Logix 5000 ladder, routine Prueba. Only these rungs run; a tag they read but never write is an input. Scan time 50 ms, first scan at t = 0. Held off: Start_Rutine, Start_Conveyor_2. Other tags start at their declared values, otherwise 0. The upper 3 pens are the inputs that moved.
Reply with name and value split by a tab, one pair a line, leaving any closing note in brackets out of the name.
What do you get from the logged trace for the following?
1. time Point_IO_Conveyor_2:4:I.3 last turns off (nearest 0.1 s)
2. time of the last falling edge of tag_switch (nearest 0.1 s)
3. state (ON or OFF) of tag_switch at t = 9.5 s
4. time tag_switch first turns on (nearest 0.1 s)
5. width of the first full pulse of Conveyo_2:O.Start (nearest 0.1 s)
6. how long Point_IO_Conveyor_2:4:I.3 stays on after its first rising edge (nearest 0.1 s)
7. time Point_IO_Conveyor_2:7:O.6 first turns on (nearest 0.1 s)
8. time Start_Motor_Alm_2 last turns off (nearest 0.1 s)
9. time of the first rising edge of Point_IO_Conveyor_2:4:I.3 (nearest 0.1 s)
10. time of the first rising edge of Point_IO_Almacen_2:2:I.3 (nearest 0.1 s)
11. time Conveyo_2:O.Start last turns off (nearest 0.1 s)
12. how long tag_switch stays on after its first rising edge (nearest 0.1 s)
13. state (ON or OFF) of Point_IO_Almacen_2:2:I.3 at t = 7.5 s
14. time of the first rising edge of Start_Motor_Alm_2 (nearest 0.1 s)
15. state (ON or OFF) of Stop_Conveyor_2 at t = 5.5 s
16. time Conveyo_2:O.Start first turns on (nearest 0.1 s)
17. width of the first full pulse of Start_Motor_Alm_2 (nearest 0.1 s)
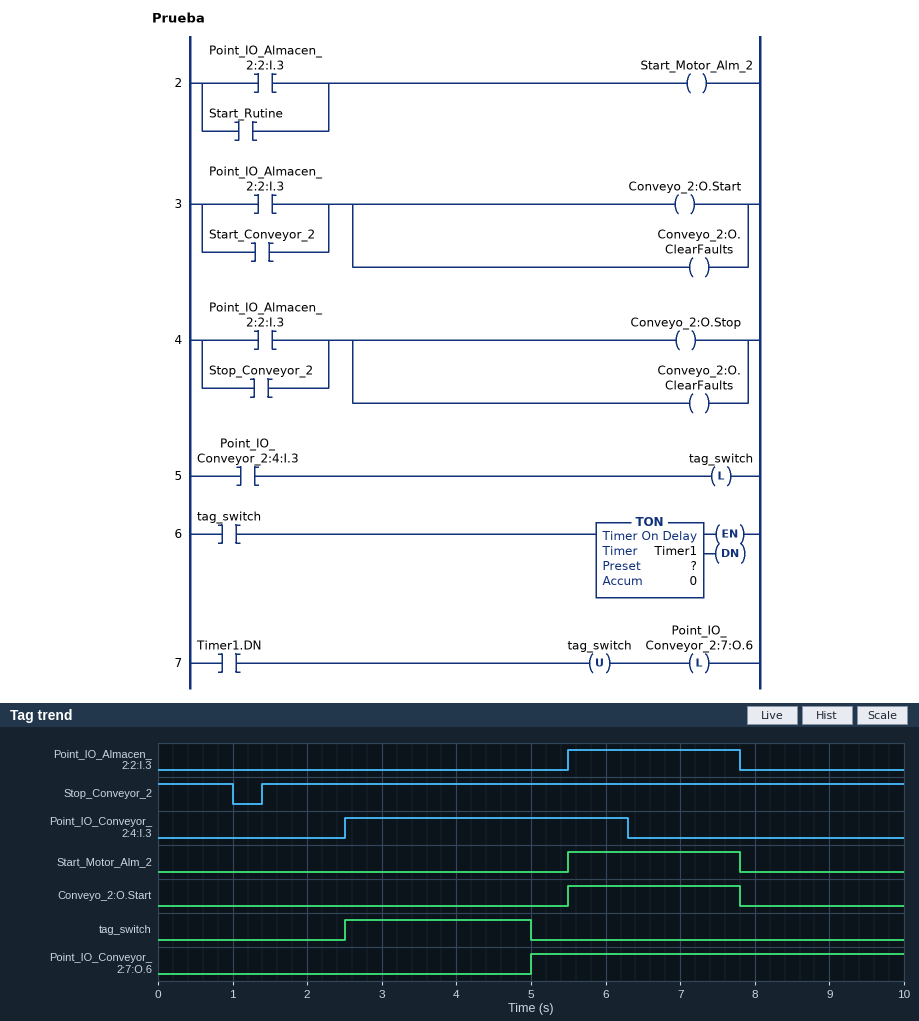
time Point_IO_Conveyor_2:4:I.3 last turns off	6.3 s
time of the last falling edge of tag_switch	5.0 s
state (ON or OFF) of tag_switch at t = 9.5 s	OFF
time tag_switch first turns on	2.5 s
width of the first full pulse of Conveyo_2:O.Start	2.3 s
how long Point_IO_Conveyor_2:4:I.3 stays on after its first rising edge	3.8 s
time Point_IO_Conveyor_2:7:O.6 first turns on	5.0 s
time Start_Motor_Alm_2 last turns off	7.8 s
time of the first rising edge of Point_IO_Conveyor_2:4:I.3	2.5 s
time of the first rising edge of Point_IO_Almacen_2:2:I.3	5.5 s
time Conveyo_2:O.Start last turns off	7.8 s
how long tag_switch stays on after its first rising edge	2.5 s
state (ON or OFF) of Point_IO_Almacen_2:2:I.3 at t = 7.5 s	ON
time of the first rising edge of Start_Motor_Alm_2	5.5 s
state (ON or OFF) of Stop_Conveyor_2 at t = 5.5 s	ON
time Conveyo_2:O.Start first turns on	5.5 s
width of the first full pulse of Start_Motor_Alm_2	2.3 s
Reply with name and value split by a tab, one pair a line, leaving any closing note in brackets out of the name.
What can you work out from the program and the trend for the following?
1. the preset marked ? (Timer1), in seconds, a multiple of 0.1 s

the preset marked ? (Timer1), in seconds, a multiple of 0.1 s	2.5 s
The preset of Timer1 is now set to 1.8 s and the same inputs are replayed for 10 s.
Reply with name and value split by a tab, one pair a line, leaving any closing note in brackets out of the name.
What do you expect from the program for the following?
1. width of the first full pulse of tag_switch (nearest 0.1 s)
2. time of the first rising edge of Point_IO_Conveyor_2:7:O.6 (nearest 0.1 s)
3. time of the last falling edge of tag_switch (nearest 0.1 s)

width of the first full pulse of tag_switch	1.8 s
time of the first rising edge of Point_IO_Conveyor_2:7:O.6	4.3 s
time of the last falling edge of tag_switch	4.3 s
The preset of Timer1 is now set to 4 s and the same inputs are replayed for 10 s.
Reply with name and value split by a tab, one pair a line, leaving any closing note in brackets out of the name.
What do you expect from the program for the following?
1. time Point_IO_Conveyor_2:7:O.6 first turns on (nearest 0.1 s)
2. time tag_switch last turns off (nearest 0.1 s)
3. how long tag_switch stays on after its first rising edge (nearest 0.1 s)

time Point_IO_Conveyor_2:7:O.6 first turns on	6.5 s
time tag_switch last turns off	6.5 s
how long tag_switch stays on after its first rising edge	4.0 s
